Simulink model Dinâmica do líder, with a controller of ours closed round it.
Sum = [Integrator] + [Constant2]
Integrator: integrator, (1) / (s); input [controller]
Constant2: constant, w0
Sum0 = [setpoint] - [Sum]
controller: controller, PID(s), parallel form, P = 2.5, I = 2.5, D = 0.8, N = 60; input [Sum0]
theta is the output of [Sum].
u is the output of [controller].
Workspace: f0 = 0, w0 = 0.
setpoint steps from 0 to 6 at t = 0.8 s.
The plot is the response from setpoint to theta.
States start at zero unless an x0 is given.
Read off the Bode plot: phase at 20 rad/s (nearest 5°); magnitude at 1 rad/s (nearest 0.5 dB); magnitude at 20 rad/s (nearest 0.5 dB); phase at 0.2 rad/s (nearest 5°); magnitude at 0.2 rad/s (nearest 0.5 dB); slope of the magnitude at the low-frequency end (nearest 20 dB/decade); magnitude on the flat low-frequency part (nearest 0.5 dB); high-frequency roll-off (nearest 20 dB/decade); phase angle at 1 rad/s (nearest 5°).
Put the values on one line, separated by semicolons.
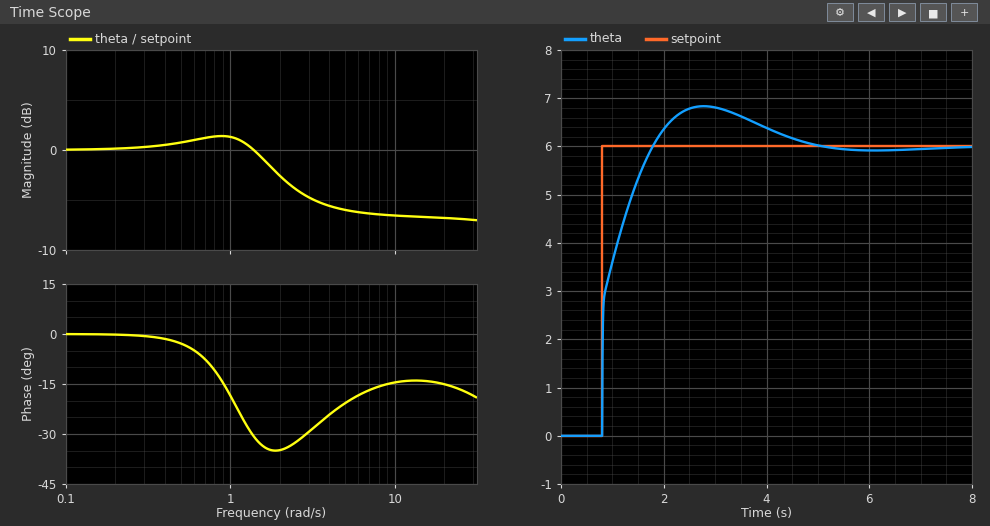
-15°; 1.5 dB; -7.0 dB; 0°; 0.0 dB; 0 dB/decade; 0.0 dB; 0 dB/decade; -20°
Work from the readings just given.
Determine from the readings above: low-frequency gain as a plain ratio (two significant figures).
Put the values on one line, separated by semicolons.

1.0
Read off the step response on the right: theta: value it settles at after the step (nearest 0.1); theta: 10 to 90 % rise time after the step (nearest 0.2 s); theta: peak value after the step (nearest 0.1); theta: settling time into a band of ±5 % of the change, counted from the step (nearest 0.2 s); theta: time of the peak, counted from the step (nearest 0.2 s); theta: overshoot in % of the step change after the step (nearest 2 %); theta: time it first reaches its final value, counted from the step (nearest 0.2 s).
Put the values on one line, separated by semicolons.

6.0; 0.8 s; 6.8; 3.4 s; 2.0 s; 14 %; 1.0 s
